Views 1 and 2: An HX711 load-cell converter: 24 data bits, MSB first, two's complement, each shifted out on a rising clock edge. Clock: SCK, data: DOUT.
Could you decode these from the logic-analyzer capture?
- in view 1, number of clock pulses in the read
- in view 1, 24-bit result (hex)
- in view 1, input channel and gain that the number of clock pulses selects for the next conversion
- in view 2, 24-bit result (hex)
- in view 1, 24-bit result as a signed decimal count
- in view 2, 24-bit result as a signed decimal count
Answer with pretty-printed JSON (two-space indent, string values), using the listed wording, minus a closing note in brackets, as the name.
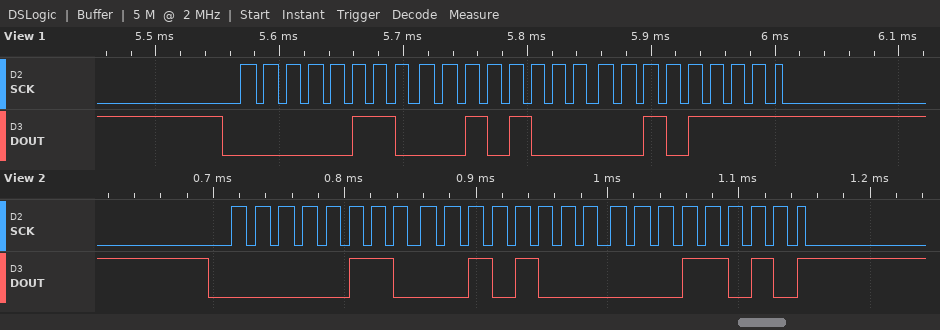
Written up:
{
  "in view 1, number of clock pulses in the read": "25",
  "in view 1, 24-bit result": "0x06282F",
  "in view 1, input channel and gain that the number of clock pulses selects for the next conversion": "channel A, gain 128",
  "in view 2, 24-bit result": "0x06281A",
  "in view 1, 24-bit result as a signed decimal count": "403503",
  "in view 2, 24-bit result as a signed decimal count": "403482"
}
